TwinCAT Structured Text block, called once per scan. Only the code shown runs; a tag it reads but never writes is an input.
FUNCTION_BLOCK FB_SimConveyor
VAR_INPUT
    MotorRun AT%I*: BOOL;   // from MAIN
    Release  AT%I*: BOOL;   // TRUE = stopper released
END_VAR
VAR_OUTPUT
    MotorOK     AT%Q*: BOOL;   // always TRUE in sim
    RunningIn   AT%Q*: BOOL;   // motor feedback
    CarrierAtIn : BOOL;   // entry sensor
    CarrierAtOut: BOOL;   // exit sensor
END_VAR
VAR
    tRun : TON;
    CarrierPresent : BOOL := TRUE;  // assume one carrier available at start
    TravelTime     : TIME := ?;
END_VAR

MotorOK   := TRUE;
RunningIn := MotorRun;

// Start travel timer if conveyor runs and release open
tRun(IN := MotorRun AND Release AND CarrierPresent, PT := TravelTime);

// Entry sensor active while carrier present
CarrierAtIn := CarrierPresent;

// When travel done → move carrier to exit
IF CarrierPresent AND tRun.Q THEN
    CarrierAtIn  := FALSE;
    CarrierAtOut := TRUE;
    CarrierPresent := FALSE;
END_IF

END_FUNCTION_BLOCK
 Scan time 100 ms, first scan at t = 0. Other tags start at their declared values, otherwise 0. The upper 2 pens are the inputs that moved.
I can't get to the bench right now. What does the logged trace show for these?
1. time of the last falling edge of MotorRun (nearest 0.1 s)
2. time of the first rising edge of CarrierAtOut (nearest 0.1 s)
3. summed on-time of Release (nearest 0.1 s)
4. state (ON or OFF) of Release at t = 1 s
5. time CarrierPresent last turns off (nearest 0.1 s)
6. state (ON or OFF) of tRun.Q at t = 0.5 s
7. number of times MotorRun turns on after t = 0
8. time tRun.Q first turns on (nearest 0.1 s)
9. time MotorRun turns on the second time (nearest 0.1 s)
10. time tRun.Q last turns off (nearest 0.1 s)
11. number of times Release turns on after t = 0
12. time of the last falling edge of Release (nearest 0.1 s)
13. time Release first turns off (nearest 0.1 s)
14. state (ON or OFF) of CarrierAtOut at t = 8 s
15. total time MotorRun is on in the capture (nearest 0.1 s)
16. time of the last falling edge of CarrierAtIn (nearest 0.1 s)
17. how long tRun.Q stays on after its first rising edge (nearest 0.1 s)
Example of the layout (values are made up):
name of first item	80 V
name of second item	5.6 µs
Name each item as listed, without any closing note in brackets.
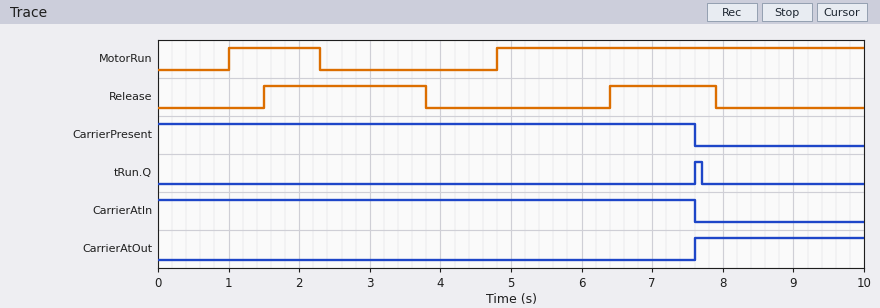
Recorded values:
time of the last falling edge of MotorRun	2.3 s
time of the first rising edge of CarrierAtOut	7.6 s
summed on-time of Release	3.8 s
state (ON or OFF) of Release at t = 1 s	OFF
time CarrierPresent last turns off	7.6 s
state (ON or OFF) of tRun.Q at t = 0.5 s	OFF
number of times MotorRun turns on after t = 0	2
time tRun.Q first turns on	7.6 s
time MotorRun turns on the second time	4.8 s
time tRun.Q last turns off	7.7 s
number of times Release turns on after t = 0	2
time of the last falling edge of Release	7.9 s
time Release first turns off	3.8 s
state (ON or OFF) of CarrierAtOut at t = 8 s	ON
total time MotorRun is on in the capture	6.5 s
time of the last falling edge of CarrierAtIn	7.6 s
how long tRun.Q stays on after its first rising edge	0.1 s
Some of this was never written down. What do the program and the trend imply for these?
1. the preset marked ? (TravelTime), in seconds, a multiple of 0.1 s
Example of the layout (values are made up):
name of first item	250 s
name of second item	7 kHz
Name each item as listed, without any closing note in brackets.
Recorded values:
the preset marked ? (TravelTime), in seconds, a multiple of 0.1 s	1.2 s
